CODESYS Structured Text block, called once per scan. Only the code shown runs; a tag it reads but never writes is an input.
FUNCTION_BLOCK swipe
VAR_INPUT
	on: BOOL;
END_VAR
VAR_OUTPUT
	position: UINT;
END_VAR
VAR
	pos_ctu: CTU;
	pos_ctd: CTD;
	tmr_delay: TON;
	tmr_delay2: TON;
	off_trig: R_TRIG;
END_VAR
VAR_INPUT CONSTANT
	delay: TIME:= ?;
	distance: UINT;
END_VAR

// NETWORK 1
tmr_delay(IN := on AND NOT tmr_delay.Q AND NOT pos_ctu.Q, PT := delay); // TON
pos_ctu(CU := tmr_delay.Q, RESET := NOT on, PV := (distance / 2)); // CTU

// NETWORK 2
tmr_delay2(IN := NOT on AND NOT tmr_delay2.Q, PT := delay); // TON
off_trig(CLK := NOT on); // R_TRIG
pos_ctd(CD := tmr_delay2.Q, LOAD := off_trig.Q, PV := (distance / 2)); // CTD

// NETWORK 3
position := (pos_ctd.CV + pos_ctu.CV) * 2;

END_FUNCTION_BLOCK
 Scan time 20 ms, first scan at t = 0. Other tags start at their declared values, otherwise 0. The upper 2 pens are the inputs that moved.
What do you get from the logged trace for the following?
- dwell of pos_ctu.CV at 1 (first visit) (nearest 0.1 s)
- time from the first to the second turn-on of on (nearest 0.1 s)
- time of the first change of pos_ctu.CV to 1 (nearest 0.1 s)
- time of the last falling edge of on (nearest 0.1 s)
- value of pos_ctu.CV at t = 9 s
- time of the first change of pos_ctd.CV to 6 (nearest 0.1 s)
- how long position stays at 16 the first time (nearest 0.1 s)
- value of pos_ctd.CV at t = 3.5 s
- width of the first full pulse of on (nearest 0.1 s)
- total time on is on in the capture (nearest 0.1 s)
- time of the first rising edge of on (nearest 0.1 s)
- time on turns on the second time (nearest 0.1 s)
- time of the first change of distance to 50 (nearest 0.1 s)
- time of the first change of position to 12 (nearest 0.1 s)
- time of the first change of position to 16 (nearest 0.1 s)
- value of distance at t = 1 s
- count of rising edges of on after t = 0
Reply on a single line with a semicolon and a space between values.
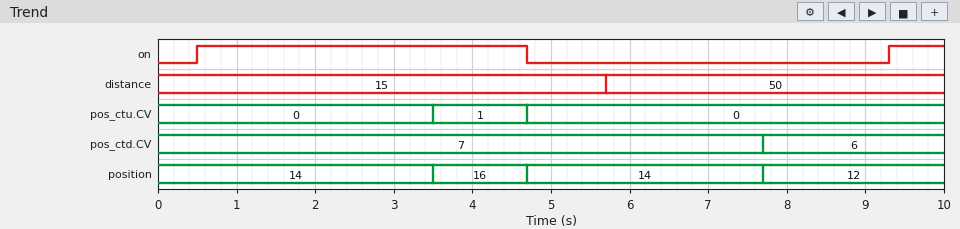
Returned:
1.2 s; 8.8 s; 3.5 s; 4.7 s; 0; 7.7 s; 1.2 s; 7; 4.2 s; 4.9 s; 0.5 s; 9.3 s; 5.7 s; 7.7 s; 3.5 s; 15; 2
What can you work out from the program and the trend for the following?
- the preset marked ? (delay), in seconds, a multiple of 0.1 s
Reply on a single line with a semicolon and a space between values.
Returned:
3.0 s
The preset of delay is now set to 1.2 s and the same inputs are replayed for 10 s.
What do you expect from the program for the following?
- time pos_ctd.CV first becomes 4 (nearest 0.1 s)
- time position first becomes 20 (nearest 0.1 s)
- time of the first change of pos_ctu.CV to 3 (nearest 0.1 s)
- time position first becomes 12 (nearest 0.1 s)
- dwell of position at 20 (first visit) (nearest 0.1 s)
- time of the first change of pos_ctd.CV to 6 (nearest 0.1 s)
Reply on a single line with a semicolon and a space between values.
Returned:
8.4 s; 4.2 s; 4.2 s; 5.9 s; 0.5 s; 5.9 s
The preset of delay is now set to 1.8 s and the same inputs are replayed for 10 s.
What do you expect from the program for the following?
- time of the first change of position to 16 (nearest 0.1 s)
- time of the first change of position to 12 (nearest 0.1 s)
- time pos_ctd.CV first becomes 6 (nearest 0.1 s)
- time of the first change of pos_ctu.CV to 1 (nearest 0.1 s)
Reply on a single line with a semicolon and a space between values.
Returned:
2.3 s; 6.5 s; 6.5 s; 2.3 s
